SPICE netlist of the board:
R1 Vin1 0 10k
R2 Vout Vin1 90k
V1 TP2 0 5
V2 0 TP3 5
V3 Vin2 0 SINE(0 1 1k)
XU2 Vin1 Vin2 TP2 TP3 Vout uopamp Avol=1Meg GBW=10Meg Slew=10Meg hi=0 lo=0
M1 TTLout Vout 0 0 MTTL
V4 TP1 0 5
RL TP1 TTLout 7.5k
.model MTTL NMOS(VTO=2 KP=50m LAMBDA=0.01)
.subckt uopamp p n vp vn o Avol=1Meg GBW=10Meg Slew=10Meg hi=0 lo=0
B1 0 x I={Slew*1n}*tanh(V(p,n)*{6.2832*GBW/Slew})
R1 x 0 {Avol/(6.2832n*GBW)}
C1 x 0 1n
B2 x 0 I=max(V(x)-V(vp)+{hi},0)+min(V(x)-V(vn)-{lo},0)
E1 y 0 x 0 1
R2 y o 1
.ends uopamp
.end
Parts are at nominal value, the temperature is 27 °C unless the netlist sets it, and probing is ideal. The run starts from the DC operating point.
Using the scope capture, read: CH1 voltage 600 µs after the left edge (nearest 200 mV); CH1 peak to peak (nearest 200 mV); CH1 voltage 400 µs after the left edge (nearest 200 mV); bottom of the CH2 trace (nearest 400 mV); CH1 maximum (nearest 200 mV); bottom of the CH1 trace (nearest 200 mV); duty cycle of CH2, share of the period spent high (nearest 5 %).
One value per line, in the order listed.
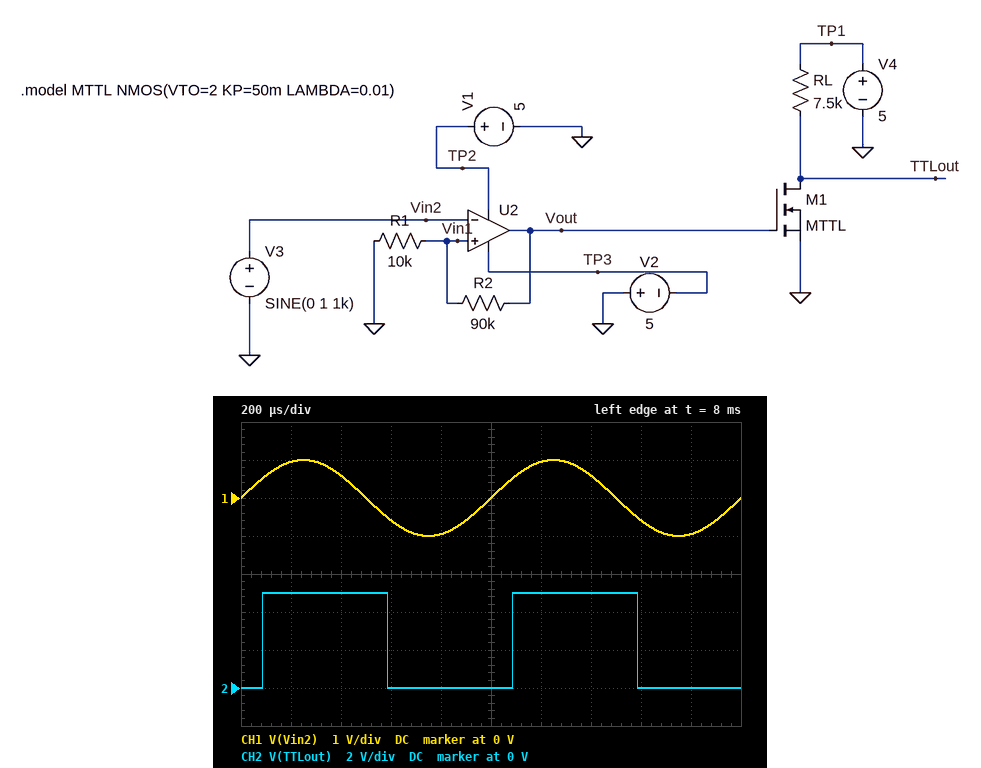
-600 mV
2.0 V
600 mV
0 V
1.0 V
-1.0 V
50 %
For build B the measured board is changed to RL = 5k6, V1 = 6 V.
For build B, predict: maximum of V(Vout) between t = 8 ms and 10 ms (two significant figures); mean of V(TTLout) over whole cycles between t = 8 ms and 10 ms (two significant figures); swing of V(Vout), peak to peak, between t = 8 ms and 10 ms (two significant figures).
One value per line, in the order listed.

6.0 V
2.4 V
11 V
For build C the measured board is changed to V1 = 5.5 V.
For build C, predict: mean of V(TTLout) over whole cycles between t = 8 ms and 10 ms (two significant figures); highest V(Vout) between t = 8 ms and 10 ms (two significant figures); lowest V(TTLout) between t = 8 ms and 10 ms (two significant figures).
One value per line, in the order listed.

2.5 V
5.5 V
3.8 mV
